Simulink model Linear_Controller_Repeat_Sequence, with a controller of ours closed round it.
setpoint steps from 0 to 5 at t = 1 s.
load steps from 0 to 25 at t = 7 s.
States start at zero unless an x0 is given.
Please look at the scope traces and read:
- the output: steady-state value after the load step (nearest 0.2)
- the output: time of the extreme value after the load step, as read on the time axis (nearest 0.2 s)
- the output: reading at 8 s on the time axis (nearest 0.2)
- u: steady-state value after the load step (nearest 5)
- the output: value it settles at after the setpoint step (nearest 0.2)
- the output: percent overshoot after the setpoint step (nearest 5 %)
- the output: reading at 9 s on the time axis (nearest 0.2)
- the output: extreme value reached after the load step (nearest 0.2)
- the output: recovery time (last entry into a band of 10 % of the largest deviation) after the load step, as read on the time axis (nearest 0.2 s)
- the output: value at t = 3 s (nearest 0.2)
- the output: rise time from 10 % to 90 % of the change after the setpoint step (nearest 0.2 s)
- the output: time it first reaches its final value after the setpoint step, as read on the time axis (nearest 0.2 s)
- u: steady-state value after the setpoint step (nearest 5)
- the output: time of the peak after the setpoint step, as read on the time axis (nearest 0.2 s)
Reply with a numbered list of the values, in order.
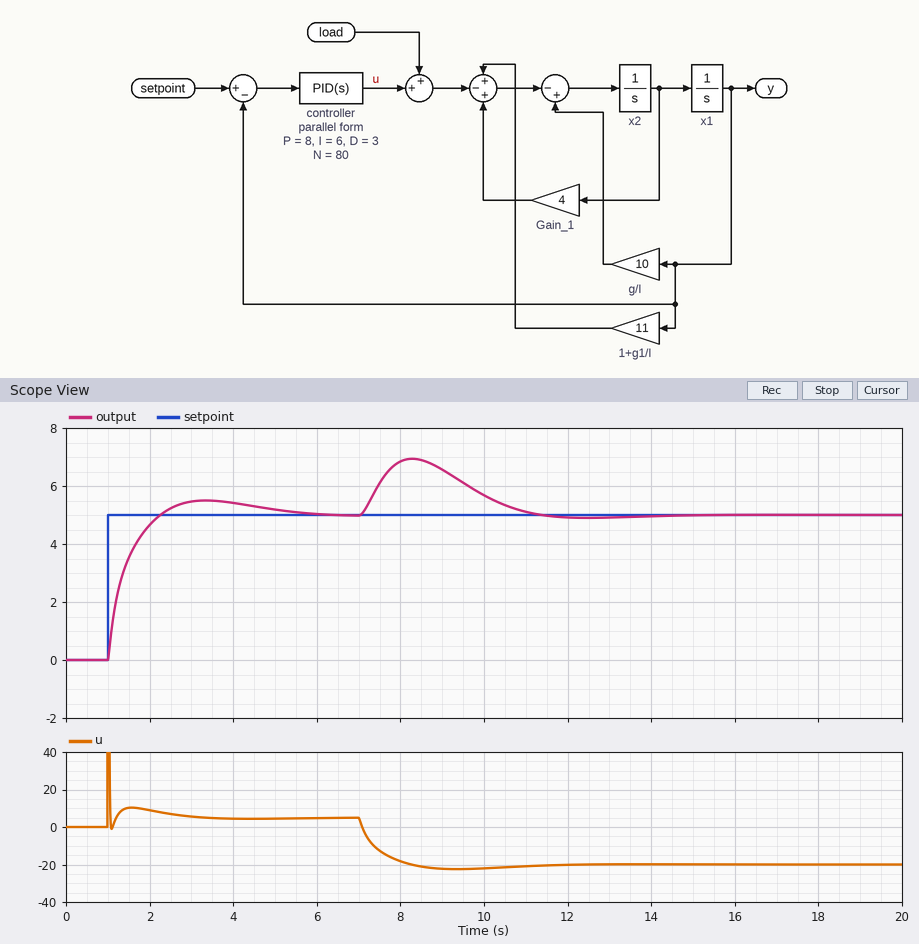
1. 5.0
2. 8.2 s
3. 6.8
4. -20
5. 5.0
6. 10 %
7. 6.6
8. 7.0
9. 10.8 s
10. 5.4
11. 0.8 s
12. 2.2 s
13. 5
14. 3.4 s
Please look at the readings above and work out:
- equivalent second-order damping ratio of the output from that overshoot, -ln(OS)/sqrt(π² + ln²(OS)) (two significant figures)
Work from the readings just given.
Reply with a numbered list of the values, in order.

1. 0.59
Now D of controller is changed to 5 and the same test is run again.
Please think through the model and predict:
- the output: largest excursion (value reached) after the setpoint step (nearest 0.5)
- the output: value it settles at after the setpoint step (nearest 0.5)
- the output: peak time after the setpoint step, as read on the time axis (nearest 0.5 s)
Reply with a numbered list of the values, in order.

1. 5.5
2. 5.0
3. 4.0 s
